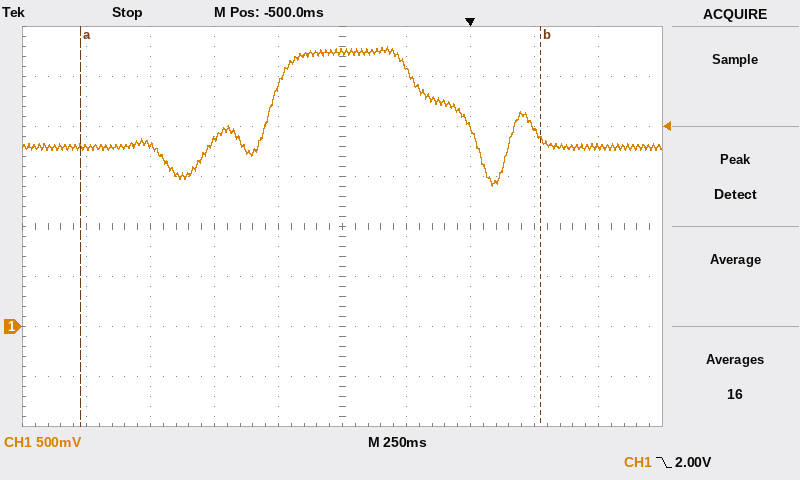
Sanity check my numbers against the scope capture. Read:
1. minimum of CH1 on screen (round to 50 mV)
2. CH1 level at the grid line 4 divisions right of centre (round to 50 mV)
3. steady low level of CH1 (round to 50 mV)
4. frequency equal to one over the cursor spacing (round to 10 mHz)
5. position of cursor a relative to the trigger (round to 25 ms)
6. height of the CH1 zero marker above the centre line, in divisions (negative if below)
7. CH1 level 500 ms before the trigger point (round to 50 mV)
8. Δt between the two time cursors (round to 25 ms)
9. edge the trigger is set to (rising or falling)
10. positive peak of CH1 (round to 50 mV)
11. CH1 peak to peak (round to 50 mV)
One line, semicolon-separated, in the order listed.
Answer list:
1.40 V; 1.80 V; 1.80 V; 560 mHz; -1.525 s; -2.0 div; 2.75 V; 1.800 s; falling; 2.80 V; 1.40 V
